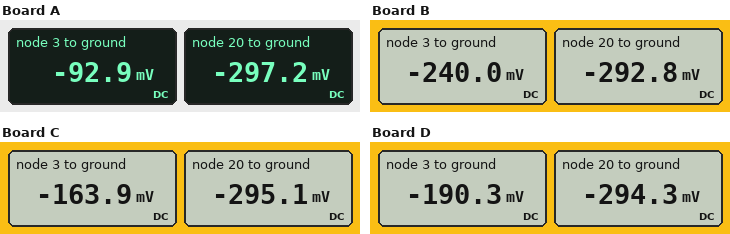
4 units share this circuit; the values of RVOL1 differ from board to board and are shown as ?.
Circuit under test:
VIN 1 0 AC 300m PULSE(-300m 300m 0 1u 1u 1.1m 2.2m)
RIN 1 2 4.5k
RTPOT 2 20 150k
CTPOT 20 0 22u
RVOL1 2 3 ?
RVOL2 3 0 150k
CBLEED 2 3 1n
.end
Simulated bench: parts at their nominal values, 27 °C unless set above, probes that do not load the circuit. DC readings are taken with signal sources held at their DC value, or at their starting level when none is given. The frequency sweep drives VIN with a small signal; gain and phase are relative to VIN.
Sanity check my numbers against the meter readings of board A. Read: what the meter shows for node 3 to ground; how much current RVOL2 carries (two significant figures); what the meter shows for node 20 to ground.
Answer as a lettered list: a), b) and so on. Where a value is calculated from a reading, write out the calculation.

a) -92.9 mV
b) (0 V - (-92.9 mV)) / 150 kΩ = 620 nA
c) -297.2 mV
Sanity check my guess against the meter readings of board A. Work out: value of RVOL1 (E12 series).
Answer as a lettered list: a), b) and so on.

a) 330 kΩ
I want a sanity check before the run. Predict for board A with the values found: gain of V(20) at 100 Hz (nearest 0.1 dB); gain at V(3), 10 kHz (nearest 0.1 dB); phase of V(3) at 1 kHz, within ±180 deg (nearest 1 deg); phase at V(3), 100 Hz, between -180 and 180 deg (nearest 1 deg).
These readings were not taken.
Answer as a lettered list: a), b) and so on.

a) -66.7 dB
b) -0.6 dB
c) 31 deg
d) 8 deg
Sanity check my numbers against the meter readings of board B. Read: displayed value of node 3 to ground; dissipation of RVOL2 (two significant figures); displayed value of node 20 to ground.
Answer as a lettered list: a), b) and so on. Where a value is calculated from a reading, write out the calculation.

a) -240.0 mV
b) (0 V - (-240 mV))^2 / 150 kΩ = 380 nW
c) -292.8 mV
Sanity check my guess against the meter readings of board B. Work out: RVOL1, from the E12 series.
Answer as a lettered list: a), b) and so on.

a) 33 kΩ
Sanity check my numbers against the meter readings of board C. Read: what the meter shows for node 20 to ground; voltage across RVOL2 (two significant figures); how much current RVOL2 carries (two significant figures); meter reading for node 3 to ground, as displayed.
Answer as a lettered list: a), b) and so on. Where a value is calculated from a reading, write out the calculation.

a) -295.1 mV
b) 0 V - (-163.9 mV) = 160 mV
c) (0 V - (-163.9 mV)) / 150 kΩ = 1.1 µA
d) -163.9 mV
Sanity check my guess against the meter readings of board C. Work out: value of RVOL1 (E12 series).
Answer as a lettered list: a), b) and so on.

a) 120 kΩ
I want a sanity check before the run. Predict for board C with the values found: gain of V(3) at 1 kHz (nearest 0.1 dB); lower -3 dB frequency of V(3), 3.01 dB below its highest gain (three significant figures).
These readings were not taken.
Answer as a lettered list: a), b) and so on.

a) -4.3 dB
b) 1.43 kHz
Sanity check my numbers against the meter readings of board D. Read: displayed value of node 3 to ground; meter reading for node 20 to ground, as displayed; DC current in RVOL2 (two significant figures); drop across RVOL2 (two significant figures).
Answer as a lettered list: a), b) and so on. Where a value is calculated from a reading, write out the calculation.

a) -190.3 mV
b) -294.3 mV
c) (0 V - (-190.3 mV)) / 150 kΩ = 1.3 µA
d) 0 V - (-190.3 mV) = 190 mV
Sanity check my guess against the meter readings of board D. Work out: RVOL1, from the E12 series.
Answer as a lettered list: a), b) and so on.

a) 82 kΩ
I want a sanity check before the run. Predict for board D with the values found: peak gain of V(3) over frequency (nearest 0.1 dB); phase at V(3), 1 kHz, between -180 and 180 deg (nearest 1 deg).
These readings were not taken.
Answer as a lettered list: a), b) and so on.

a) -0.5 dB
b) 9 deg
